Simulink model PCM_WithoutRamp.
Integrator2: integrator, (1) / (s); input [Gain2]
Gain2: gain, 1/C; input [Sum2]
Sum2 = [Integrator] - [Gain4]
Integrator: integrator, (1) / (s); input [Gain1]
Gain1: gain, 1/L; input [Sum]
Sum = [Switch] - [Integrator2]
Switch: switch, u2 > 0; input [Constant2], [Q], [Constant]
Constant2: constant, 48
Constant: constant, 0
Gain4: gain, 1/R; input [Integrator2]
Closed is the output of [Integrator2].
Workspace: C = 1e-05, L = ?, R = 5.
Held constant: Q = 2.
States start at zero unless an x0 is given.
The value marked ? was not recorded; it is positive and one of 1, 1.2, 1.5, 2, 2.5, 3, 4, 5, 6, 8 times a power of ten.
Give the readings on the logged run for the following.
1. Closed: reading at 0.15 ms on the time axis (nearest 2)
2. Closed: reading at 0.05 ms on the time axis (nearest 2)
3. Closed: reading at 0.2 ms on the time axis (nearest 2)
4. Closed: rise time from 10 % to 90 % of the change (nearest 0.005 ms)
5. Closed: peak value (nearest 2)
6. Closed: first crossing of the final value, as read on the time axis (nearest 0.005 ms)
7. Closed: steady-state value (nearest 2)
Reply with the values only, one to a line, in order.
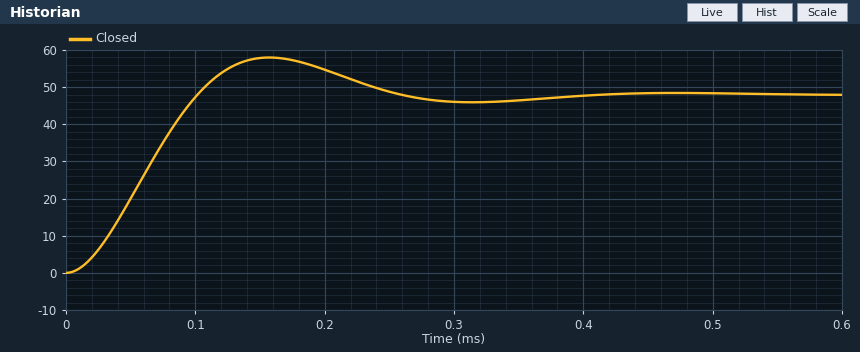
58
20
54
0.070 ms
58
0.100 ms
48
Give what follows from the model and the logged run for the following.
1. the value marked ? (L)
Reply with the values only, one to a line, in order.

0.0002
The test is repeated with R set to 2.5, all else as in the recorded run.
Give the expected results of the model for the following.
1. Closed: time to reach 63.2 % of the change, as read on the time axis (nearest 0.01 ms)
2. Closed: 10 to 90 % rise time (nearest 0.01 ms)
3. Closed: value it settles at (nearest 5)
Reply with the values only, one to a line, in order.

0.09 ms
0.13 ms
50
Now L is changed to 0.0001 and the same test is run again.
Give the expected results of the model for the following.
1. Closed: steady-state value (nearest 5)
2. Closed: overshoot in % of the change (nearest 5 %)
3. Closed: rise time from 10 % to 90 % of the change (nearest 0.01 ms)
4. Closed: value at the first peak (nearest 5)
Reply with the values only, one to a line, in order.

50
35 %
0.04 ms
65
